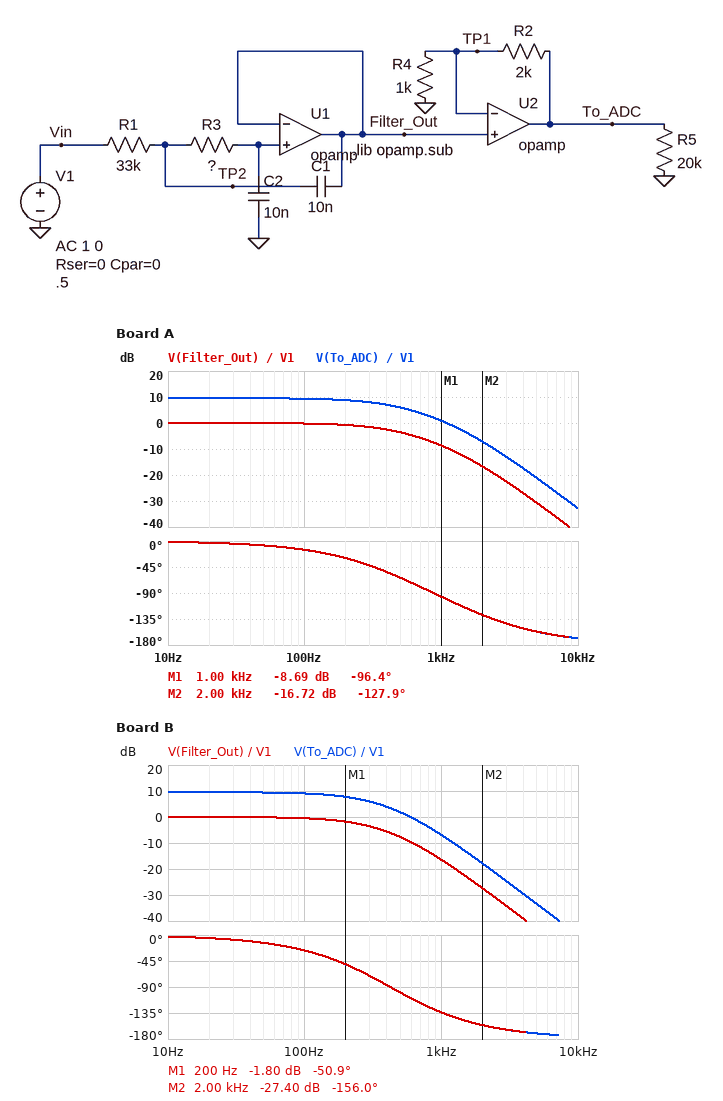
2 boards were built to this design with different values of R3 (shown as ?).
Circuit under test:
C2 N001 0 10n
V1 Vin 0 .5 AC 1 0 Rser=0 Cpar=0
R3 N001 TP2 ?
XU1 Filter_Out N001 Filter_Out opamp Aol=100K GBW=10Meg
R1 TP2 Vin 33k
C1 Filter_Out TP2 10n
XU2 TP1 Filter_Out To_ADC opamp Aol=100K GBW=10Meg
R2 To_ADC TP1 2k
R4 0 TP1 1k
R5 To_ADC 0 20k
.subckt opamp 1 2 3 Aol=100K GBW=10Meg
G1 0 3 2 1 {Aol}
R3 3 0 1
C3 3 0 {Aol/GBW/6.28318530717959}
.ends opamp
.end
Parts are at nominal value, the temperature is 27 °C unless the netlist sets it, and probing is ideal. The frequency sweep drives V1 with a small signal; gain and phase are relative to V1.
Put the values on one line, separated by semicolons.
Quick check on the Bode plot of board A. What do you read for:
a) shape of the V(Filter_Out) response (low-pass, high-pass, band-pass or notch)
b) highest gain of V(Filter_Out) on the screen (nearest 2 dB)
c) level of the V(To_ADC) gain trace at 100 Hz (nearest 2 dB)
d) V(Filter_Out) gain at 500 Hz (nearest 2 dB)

low-pass; 0 dB; 10 dB; -4 dB
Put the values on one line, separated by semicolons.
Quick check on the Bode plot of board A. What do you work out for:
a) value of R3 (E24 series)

10 kΩ
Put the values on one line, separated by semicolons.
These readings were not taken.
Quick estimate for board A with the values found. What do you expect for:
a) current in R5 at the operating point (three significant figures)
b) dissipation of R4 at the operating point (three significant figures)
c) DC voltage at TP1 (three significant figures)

75.0 µA; 250 µW; 500 mV
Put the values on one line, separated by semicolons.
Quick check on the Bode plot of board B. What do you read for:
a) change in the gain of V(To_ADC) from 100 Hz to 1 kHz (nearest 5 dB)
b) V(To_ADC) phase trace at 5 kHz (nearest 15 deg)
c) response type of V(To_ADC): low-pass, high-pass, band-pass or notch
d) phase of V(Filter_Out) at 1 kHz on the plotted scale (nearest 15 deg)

-15 dB; -165 deg; low-pass; -135 deg
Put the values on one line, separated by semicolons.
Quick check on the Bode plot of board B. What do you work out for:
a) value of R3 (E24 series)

43 kΩ
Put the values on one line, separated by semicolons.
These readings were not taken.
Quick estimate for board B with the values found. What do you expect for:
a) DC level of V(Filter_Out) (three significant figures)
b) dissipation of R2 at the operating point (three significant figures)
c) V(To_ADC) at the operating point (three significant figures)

500 mV; 500 µW; 1.50 V
